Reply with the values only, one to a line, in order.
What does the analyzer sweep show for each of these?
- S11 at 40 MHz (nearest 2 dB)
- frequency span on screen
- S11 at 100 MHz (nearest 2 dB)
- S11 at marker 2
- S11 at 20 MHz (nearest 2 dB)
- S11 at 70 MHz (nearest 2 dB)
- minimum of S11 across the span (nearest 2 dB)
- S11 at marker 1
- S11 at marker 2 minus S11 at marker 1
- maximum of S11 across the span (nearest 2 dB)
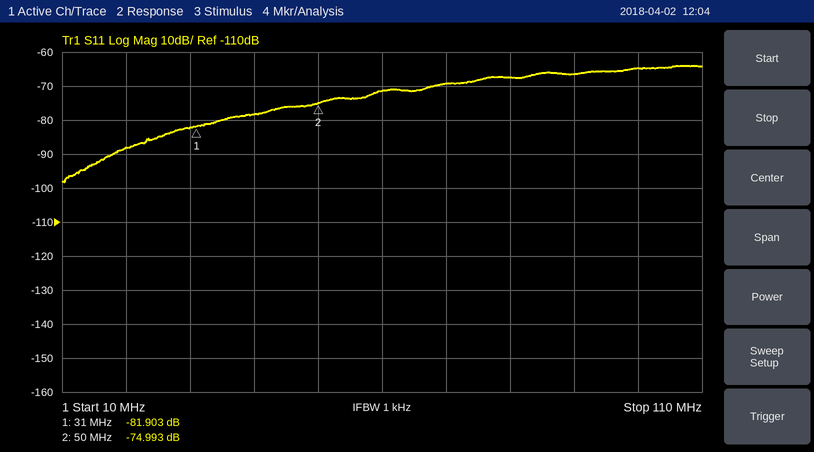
-78 dB
100 MHz
-64 dB
-74.993 dB
-88 dB
-70 dB
-98 dB
-81.903 dB
6.910 dB
-64 dB
